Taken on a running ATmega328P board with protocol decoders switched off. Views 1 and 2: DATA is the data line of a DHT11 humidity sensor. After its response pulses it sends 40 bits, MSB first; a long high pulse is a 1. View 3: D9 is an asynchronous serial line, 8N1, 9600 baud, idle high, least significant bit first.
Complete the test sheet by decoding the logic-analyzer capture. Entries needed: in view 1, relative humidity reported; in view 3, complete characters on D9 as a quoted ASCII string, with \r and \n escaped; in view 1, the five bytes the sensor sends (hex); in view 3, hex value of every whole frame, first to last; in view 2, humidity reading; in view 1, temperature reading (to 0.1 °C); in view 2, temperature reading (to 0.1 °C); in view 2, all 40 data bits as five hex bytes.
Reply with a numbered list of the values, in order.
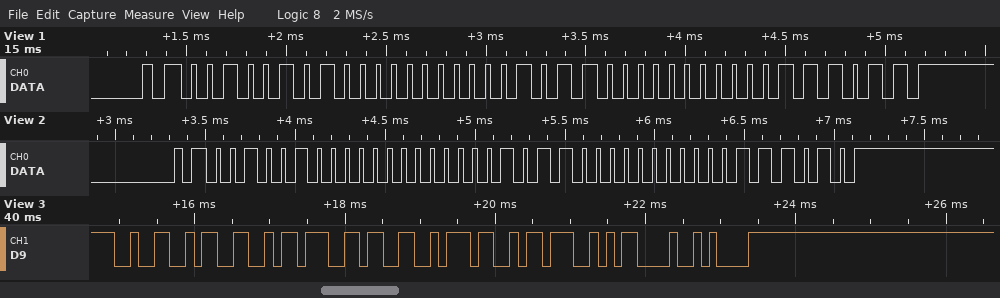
1. 37 %
2. "23;37;\r\n"
3. 25 00 16 00 3B
4. 32 33 3B 33 37 3B 0D 0A
5. 36 %
6. 22.0 °C
7. 22.0 °C
8. 24 00 16 00 3A
